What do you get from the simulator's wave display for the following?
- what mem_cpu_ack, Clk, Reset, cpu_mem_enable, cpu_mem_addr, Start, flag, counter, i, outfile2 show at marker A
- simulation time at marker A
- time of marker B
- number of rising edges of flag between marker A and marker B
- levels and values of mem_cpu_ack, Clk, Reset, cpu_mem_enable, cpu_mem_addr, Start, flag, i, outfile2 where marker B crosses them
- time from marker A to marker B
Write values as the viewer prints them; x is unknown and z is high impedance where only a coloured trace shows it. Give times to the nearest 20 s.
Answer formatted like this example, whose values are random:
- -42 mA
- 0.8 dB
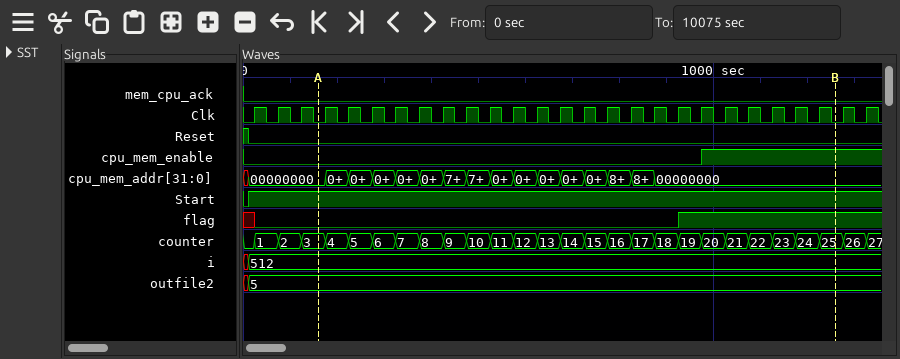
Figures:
- mem_cpu_ack=0, Clk=0, Reset=0, cpu_mem_enable=0, cpu_mem_addr=00000000, Start=1, flag=0, counter=3, i=512, outfile2=5
- 160 s
- 1260 s
- 1
- mem_cpu_ack=0, Clk=0, Reset=0, cpu_mem_enable=1, cpu_mem_addr=00000000, Start=1, flag=1, i=512, outfile2=5
- 1100 s
